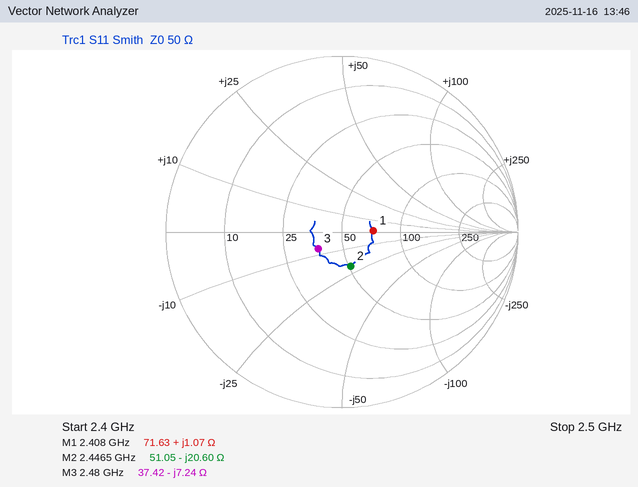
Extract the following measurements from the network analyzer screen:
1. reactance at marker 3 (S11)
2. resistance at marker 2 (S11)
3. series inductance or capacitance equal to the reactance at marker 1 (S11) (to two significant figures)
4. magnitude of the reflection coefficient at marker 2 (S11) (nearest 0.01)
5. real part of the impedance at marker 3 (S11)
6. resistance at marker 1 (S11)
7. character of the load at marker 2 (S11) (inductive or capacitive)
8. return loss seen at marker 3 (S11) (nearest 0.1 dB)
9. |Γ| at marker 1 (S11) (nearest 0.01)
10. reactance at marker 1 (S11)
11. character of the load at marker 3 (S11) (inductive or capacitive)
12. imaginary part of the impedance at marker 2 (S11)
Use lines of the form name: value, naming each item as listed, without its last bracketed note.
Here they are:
reactance at marker 3: -7.24 Ω
resistance at marker 2: 51.05 Ω
series inductance or capacitance equal to the reactance at marker 1 (S11): 71 pH
magnitude of the reflection coefficient at marker 2 (S11): 0.20
real part of the impedance at marker 3: 37.42 Ω
resistance at marker 1: 71.63 Ω
character of the load at marker 2 (S11): capacitive
return loss seen at marker 3 (S11): 15.6 dB
|Γ| at marker 1 (S11): 0.18
reactance at marker 1: +1.07 Ω
character of the load at marker 3 (S11): capacitive
imaginary part of the impedance at marker 2: -20.60 Ω
